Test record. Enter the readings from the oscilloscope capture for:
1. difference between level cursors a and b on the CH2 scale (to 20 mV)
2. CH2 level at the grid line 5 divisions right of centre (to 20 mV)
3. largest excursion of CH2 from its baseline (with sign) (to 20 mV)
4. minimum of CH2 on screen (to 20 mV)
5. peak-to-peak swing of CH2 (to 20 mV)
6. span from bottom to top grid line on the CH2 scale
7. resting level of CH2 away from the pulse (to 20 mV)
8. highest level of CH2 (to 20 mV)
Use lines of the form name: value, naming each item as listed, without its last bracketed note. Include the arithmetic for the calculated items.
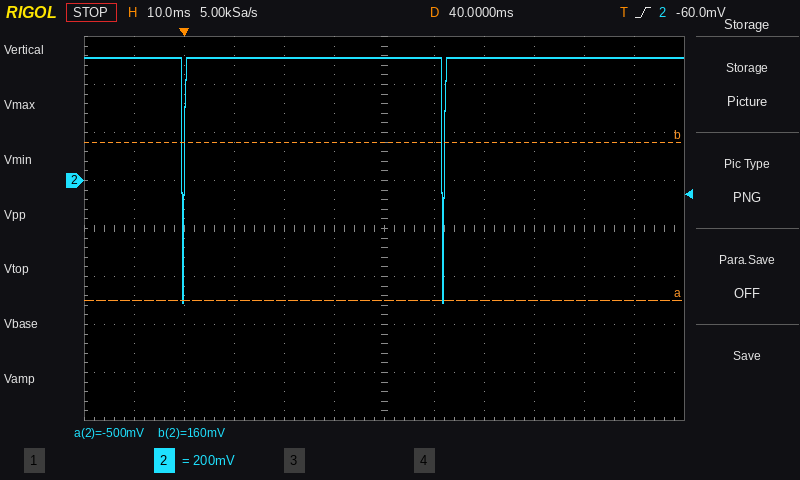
difference between level cursors a and b on the CH2 scale: 660 mV
CH2 level at the grid line 5 divisions right of centre: 520 mV
largest excursion of CH2 from its baseline (with sign): -500 mV − (520 mV) = -1.02 V
minimum of CH2 on screen: -500 mV
peak-to-peak swing of CH2: 520 mV − (-500 mV) = 1.02 V
span from bottom to top grid line on the CH2 scale: 1.6 V
resting level of CH2 away from the pulse: 520 mV
highest level of CH2: 520 mV
